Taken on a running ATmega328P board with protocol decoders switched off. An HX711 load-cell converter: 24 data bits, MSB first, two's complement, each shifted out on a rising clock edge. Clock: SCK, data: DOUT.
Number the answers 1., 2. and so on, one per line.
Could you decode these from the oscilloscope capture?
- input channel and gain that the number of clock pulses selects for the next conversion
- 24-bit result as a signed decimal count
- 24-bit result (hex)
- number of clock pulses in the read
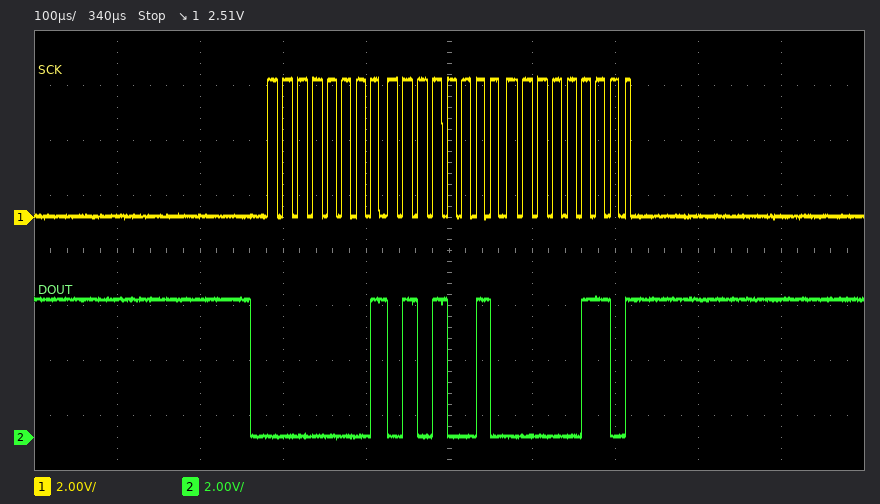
1. channel A, gain 128
2. 86534
3. 0x015206
4. 25
